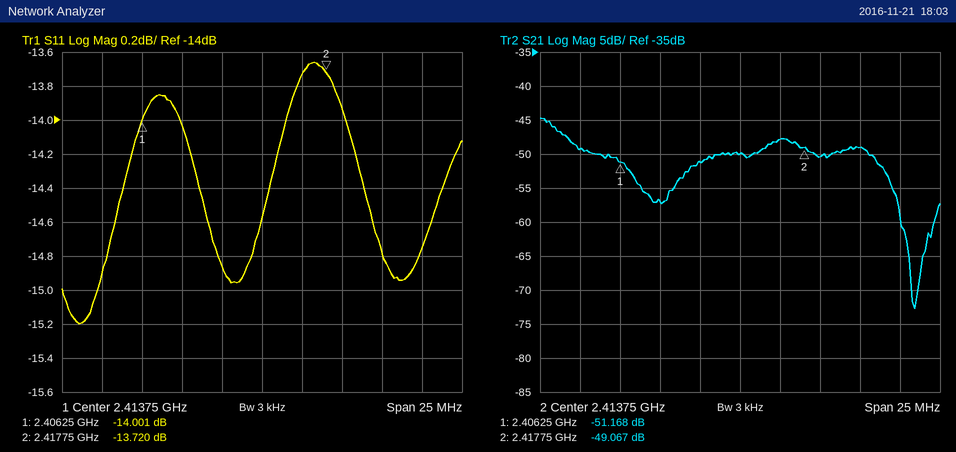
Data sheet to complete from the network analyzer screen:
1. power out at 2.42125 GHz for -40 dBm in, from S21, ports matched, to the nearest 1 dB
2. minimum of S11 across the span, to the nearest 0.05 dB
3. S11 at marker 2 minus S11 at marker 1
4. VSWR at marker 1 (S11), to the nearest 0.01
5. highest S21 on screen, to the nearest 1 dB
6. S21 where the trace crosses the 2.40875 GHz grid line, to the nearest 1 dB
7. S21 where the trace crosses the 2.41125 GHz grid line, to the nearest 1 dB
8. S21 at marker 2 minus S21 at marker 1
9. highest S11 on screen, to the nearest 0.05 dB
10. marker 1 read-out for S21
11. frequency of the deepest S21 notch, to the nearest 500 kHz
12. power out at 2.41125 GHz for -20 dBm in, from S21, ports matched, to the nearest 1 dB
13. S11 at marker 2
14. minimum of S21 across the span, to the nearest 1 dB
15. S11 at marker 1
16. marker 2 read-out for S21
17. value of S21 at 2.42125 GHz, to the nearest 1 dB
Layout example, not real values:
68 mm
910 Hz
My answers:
-89 dBm
-15.20 dB
0.281 dB
1.50
-45 dB
-57 dB
-51 dB
2.101 dB
-13.65 dB
-51.168 dB
2.4245 GHz
-71 dBm
-13.720 dB
-73 dB
-14.001 dB
-49.067 dB
-49 dB
